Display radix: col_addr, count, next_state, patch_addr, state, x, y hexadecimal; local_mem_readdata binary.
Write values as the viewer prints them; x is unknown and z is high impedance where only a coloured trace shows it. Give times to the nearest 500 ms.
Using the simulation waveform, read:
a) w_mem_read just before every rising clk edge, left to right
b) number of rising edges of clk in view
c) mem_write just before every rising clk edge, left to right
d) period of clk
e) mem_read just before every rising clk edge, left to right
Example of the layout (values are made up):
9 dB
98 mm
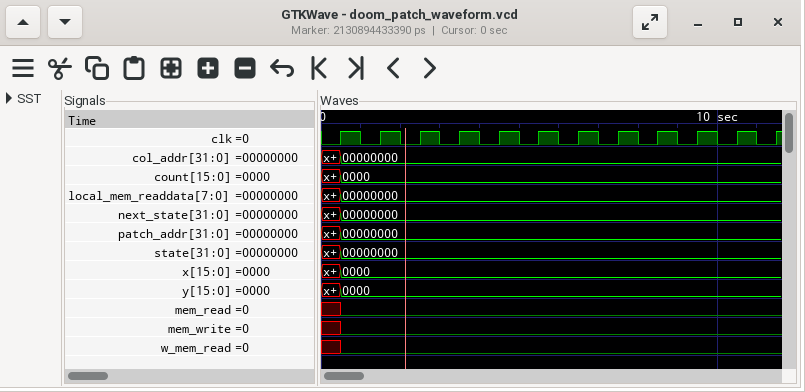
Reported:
x 0 0 0 0 0 0 0 0 0 0 0
12
x 0 0 0 0 0 0 0 0 0 0 0
1000 ms
x 0 0 0 0 0 0 0 0 0 0 0
